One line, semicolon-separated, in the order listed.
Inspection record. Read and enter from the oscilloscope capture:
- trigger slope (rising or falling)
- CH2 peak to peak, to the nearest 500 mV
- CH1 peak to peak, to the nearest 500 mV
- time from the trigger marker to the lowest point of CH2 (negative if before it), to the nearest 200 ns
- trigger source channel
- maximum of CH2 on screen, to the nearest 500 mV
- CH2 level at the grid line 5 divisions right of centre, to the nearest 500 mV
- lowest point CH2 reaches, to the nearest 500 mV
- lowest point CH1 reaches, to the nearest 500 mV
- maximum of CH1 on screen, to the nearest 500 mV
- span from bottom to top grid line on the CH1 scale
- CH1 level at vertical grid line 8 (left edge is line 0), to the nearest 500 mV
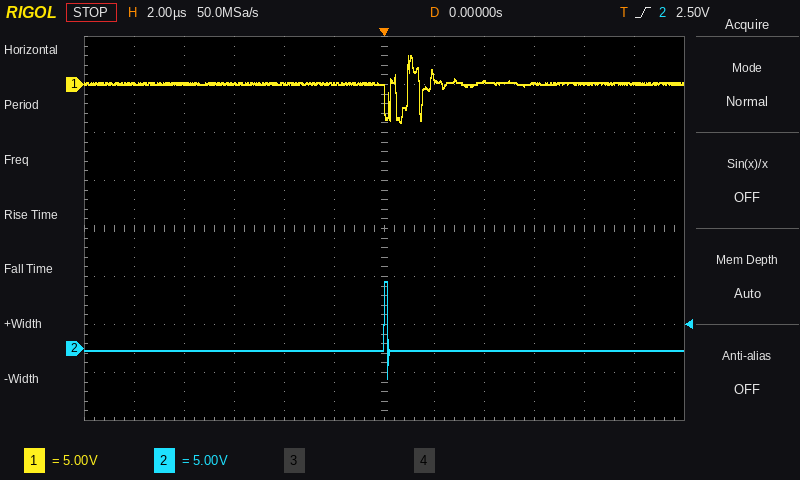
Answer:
rising; 10.0 V; 7.0 V; +200 ns; CH2; 7.0 V; 0.0 V; -3.0 V; -4.0 V; 3.0 V; 40 V; 500 mV
